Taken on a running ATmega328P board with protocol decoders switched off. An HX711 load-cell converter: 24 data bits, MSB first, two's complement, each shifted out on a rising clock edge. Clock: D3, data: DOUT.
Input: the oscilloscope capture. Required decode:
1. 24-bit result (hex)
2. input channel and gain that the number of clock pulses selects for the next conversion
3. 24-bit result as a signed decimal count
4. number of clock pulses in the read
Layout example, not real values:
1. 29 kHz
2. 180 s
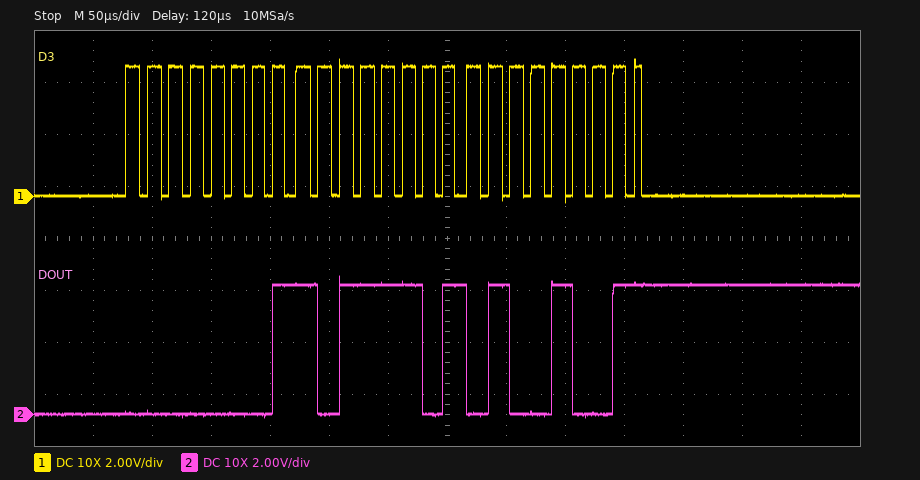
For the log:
1. 0x01BD49
2. channel A, gain 128
3. 113993
4. 25
